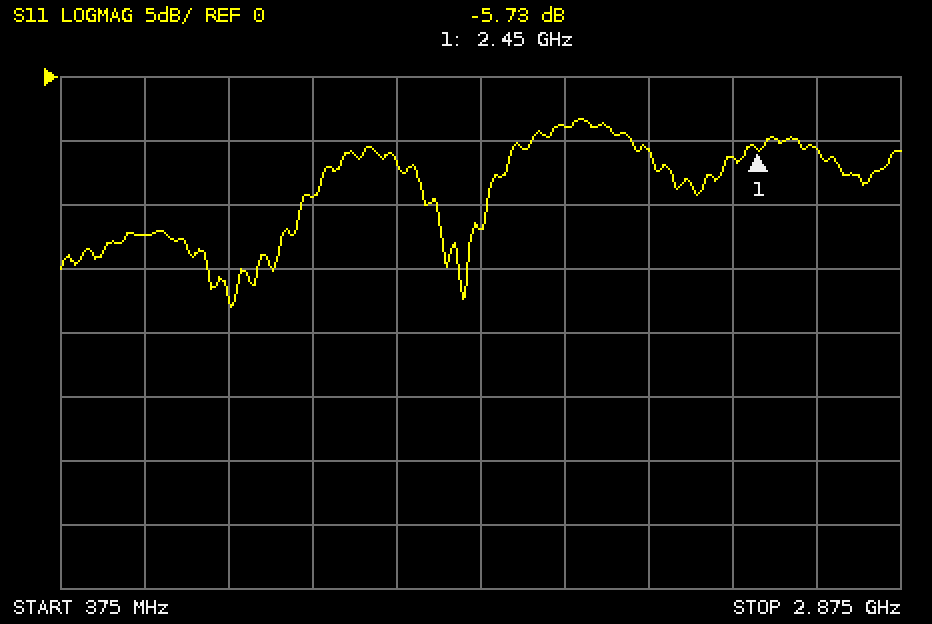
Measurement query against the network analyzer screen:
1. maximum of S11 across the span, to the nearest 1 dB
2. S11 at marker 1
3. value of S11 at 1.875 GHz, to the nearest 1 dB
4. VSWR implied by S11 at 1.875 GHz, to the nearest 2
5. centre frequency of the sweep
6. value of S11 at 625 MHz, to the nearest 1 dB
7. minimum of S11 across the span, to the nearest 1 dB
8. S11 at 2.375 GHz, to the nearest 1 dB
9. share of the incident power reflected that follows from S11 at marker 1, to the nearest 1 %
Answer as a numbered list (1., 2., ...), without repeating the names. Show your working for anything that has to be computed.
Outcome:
1. -3 dB
2. -5.73 dB
3. -4 dB
4. |Γ| = 10^(-4/20) = 0.6310; VSWR = (1 + 0.6310)/(1 − 0.6310) ≈ 4
5. 1.625 GHz
6. -12 dB
7. -18 dB
8. -6 dB
9. 10^(-5.73/10) ≈ 27 %
